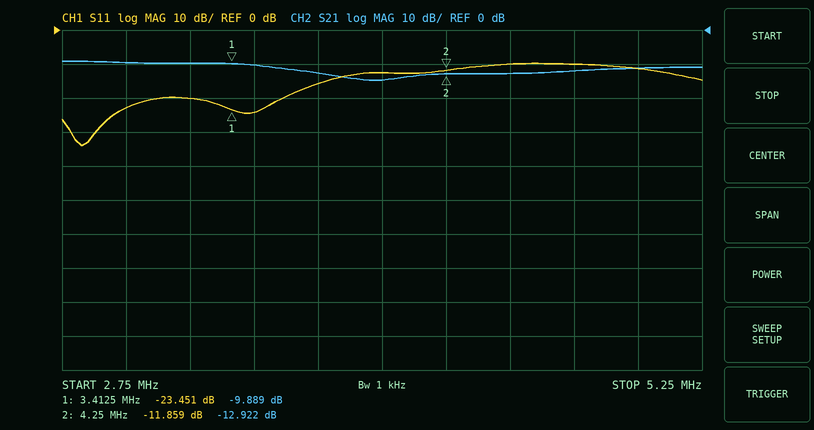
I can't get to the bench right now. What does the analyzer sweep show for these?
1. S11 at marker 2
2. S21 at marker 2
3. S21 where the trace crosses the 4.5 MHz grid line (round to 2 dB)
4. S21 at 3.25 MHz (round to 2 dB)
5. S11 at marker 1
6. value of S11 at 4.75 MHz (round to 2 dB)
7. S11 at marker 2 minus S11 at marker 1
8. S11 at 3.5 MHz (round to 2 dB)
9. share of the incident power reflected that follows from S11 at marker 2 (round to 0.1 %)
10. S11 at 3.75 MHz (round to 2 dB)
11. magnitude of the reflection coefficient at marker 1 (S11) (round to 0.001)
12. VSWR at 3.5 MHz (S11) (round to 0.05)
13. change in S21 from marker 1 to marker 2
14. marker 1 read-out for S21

-11.859 dB
-12.922 dB
-12 dB
-10 dB
-23.451 dB
-10 dB
11.592 dB
-24 dB
6.5 %
-16 dB
0.067
1.15
-3.033 dB
-9.889 dB
